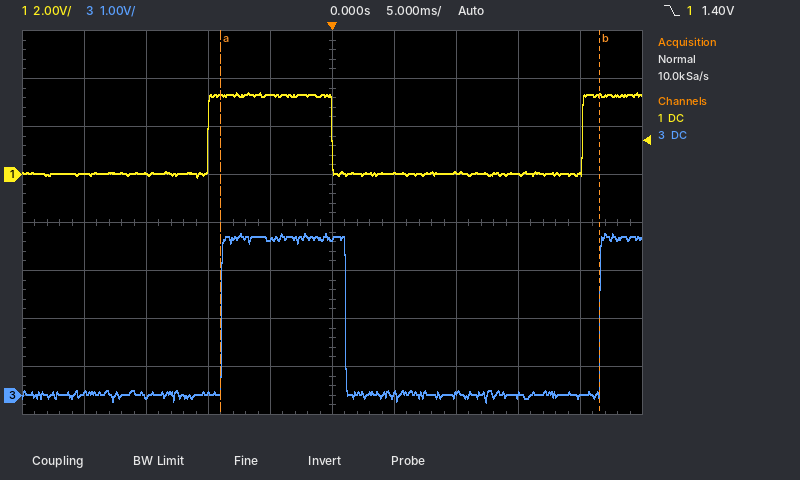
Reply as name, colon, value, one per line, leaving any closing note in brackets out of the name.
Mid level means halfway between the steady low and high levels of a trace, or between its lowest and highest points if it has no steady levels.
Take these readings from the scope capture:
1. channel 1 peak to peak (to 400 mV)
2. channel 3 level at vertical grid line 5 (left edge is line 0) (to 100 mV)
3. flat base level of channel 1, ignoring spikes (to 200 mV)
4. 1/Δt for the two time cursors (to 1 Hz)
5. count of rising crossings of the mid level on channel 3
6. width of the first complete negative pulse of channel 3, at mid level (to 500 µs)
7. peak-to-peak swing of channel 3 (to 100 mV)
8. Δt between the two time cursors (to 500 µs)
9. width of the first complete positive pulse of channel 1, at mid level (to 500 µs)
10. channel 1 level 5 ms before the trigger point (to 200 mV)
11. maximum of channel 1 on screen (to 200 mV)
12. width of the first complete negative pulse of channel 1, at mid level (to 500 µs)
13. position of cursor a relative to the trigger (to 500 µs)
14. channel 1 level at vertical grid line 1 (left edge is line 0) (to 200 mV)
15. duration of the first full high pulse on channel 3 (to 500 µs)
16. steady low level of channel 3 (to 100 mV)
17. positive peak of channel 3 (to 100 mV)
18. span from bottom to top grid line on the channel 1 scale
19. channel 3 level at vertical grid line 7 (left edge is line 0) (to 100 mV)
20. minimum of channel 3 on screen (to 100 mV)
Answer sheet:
channel 1 peak to peak: 3.6 V
channel 3 level at vertical grid line 5 (left edge is line 0): 3.3 V
flat base level of channel 1, ignoring spikes: 0.0 V
1/Δt for the two time cursors: 33 Hz
count of rising crossings of the mid level on channel 3: 2
width of the first complete negative pulse of channel 3, at mid level: 20.5 ms
peak-to-peak swing of channel 3: 3.5 V
Δt between the two time cursors: 30.5 ms
width of the first complete positive pulse of channel 1, at mid level: 10.0 ms
channel 1 level 5 ms before the trigger point: 3.4 V
maximum of channel 1 on screen: 3.4 V
width of the first complete negative pulse of channel 1, at mid level: 20.0 ms
position of cursor a relative to the trigger: -9.0 ms
channel 1 level at vertical grid line 1 (left edge is line 0): 0.0 V
duration of the first full high pulse on channel 3: 10.0 ms
steady low level of channel 3: 0.0 V
positive peak of channel 3: 3.4 V
span from bottom to top grid line on the channel 1 scale: 16 V
channel 3 level at vertical grid line 7 (left edge is line 0): 0.0 V
minimum of channel 3 on screen: -100 mV
